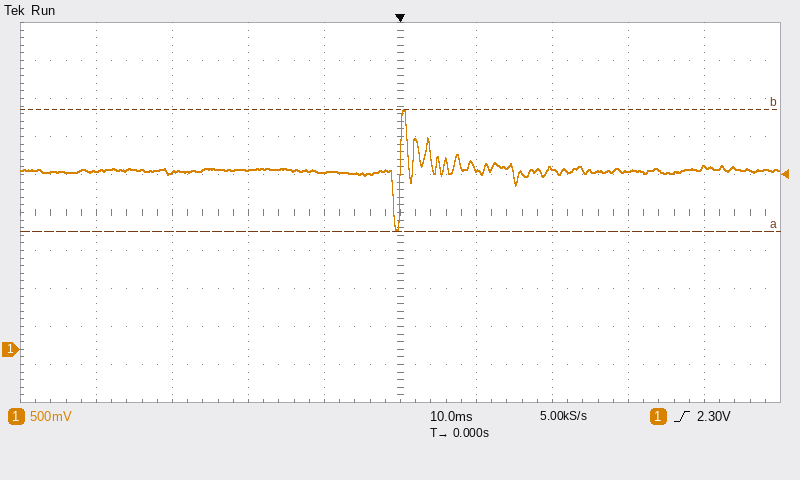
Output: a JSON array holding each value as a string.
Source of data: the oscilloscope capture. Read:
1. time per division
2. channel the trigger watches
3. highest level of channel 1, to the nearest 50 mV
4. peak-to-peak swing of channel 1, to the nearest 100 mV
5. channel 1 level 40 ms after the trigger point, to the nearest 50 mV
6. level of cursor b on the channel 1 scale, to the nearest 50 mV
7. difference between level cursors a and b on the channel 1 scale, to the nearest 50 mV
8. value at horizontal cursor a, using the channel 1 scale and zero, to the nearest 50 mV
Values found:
["10 ms", "channel 1", "3.15 V", "1.60 V", "2.40 V", "3.15 V", "1.60 V", "1.55 V"]
